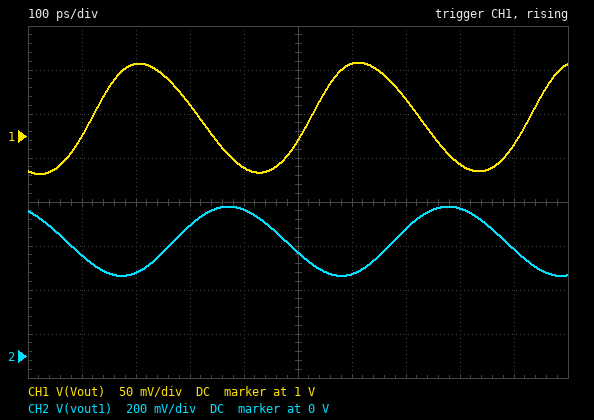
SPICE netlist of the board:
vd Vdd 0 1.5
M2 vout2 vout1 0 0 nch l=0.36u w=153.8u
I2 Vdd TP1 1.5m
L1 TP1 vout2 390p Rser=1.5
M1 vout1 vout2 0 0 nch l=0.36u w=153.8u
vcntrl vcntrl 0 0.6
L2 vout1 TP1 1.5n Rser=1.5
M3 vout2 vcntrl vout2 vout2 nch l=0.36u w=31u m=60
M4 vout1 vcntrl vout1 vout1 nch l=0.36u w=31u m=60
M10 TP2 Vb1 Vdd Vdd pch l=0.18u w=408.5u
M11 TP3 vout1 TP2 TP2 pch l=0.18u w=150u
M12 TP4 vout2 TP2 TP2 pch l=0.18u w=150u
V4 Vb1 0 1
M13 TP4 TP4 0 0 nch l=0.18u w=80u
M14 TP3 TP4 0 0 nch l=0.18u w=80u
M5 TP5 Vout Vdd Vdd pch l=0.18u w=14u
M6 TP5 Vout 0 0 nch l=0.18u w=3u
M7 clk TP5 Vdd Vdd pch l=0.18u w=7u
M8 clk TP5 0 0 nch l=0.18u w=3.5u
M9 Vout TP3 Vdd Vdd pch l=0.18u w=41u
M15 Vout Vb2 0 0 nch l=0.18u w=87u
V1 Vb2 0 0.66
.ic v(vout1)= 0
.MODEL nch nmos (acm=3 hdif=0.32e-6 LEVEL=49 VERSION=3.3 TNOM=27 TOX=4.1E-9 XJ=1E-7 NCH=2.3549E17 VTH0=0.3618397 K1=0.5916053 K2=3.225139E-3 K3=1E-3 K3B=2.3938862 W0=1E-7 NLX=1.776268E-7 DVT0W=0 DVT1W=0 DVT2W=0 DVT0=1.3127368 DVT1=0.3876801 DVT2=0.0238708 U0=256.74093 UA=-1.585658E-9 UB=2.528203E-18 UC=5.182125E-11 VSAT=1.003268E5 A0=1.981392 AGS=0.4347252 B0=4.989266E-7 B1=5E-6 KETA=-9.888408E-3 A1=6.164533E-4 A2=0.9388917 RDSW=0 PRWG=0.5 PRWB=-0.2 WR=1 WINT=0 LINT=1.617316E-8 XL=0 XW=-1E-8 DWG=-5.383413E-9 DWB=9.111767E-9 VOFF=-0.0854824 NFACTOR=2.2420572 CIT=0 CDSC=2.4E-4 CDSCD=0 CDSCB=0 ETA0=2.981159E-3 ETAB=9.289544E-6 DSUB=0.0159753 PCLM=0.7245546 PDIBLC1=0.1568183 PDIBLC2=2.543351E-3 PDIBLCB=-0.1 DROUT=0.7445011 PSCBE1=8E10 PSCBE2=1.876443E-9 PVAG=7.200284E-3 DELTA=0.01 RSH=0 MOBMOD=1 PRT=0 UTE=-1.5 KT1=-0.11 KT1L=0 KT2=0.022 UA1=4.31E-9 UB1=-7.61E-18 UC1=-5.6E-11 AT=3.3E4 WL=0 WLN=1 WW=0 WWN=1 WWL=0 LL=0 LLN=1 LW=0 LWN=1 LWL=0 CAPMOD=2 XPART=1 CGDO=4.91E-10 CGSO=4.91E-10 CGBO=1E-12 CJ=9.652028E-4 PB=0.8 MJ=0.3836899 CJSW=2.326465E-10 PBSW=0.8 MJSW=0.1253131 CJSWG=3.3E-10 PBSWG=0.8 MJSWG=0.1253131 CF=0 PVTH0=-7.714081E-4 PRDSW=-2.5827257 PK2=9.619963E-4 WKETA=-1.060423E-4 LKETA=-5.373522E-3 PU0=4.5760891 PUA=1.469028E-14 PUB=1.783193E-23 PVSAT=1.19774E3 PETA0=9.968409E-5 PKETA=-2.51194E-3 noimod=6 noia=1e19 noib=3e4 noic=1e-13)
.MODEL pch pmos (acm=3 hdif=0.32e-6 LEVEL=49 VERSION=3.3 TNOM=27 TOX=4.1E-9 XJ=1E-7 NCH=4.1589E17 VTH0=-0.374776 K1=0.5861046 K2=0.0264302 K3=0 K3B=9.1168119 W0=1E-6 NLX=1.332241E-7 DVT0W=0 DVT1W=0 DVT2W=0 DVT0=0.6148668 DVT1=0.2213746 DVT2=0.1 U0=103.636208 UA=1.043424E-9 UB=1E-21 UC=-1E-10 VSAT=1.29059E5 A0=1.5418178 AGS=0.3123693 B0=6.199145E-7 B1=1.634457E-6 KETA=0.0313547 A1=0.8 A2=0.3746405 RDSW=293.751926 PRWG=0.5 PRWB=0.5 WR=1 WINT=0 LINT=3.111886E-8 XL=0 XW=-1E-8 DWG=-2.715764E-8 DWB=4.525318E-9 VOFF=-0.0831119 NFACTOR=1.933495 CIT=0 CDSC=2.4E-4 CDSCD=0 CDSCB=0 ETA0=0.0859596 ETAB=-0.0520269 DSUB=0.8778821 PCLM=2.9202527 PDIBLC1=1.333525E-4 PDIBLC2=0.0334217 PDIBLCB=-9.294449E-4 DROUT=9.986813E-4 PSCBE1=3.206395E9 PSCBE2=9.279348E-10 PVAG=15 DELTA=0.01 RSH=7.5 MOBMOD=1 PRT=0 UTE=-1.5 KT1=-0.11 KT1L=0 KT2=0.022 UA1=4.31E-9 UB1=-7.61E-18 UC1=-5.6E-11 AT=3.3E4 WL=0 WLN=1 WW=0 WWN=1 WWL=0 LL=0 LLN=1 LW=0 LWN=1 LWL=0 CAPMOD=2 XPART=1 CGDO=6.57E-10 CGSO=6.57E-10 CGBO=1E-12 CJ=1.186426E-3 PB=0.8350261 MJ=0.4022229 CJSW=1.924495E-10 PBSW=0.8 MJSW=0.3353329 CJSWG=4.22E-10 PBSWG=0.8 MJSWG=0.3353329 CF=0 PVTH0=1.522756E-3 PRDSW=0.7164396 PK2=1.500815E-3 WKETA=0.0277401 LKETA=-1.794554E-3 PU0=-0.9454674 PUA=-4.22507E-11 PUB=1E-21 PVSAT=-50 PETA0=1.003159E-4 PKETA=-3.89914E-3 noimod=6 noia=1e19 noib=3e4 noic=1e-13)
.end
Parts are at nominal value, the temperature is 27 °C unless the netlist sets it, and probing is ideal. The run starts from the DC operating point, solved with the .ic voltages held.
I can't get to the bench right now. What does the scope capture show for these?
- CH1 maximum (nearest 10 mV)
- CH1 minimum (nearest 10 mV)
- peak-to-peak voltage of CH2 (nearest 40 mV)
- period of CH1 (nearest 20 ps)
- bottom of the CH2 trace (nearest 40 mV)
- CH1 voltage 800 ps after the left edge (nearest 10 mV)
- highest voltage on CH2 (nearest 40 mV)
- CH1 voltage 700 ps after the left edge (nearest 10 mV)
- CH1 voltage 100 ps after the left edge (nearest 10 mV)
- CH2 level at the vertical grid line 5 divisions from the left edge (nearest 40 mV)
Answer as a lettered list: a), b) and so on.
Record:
a) 1.08 V
b) 960 mV
c) 320 mV
d) 400 ps
e) 360 mV
f) 970 mV
g) 680 mV
h) 1.04 V
i) 1.00 V
j) 480 mV
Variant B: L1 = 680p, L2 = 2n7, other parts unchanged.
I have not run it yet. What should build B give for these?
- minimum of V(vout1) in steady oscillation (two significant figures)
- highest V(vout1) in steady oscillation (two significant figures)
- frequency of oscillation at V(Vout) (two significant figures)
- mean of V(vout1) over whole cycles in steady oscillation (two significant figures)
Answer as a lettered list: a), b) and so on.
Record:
a) 120 mV
b) 730 mV
c) 1.8 GHz
d) 420 mV
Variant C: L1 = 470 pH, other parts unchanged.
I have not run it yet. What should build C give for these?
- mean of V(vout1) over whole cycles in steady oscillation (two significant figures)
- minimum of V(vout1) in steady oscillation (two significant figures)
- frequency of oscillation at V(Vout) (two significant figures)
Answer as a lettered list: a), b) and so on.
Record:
a) 520 mV
b) 350 mV
c) 2.4 GHz
